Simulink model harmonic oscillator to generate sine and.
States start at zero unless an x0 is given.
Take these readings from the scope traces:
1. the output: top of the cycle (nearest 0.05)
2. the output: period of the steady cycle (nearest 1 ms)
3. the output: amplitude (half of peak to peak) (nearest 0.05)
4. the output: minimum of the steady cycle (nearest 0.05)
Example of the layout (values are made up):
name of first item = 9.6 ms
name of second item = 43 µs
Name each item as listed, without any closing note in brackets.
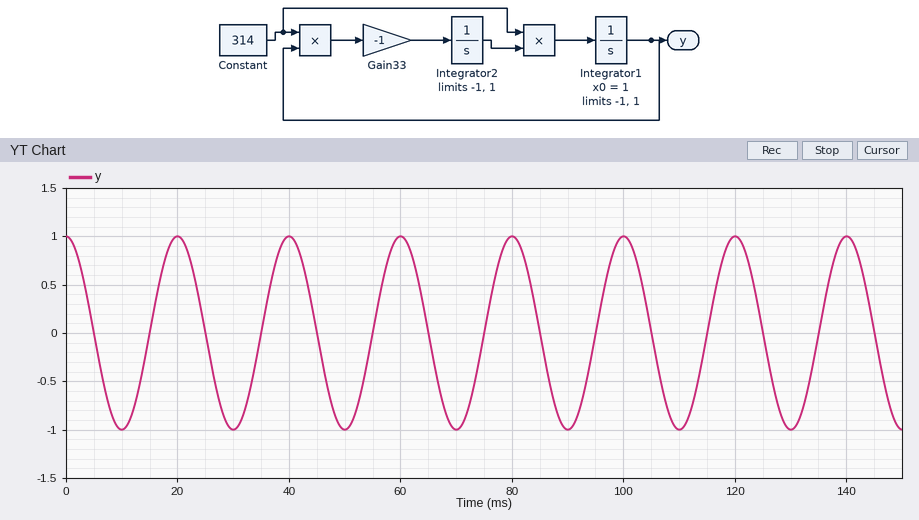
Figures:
the output: top of the cycle = 1.00
the output: period of the steady cycle = 20 ms
the output: amplitude (half of peak to peak) = 1.00
the output: minimum of the steady cycle = -1.00
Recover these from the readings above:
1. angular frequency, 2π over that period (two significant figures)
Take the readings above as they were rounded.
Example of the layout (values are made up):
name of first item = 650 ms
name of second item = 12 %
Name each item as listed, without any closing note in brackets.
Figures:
angular frequency, 2π over that period = 0.31 rad/ms
